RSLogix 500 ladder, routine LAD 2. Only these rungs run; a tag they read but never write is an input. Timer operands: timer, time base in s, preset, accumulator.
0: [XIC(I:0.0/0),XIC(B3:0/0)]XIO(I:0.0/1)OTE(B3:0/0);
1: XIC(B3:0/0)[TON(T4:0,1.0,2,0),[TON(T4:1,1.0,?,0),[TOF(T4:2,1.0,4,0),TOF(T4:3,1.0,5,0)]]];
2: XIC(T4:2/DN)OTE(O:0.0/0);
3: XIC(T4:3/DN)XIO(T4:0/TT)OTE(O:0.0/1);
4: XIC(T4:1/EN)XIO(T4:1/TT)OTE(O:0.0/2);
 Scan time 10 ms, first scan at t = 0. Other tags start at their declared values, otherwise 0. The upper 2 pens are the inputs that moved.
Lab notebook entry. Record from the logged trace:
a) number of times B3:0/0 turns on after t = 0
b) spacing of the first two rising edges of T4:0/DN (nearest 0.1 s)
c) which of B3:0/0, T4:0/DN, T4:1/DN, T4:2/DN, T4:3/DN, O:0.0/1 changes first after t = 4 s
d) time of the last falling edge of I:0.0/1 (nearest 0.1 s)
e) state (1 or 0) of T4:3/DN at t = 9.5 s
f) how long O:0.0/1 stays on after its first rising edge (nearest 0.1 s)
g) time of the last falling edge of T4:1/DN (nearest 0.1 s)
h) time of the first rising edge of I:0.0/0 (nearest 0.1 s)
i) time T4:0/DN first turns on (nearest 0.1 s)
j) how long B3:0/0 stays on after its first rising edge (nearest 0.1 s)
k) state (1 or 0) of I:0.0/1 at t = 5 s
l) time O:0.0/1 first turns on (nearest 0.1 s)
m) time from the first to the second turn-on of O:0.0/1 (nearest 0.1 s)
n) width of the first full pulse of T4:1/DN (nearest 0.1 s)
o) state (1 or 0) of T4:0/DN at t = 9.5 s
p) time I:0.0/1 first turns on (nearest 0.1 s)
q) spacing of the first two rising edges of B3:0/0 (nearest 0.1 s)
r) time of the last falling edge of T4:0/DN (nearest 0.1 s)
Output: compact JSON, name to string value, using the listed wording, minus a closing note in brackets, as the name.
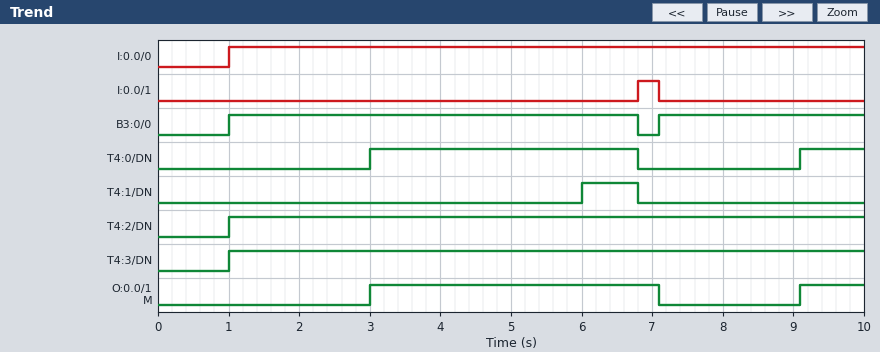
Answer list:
{"number of times B3:0/0 turns on after t = 0": "2", "spacing of the first two rising edges of T4:0/DN": "6.1 s", "which of B3:0/0, T4:0/DN, T4:1/DN, T4:2/DN, T4:3/DN, O:0.0/1 changes first after t = 4 s": "T4:1/DN", "time of the last falling edge of I:0.0/1": "7.1 s", "state (1 or 0) of T4:3/DN at t = 9.5 s": "1", "how long O:0.0/1 stays on after its first rising edge": "4.1 s", "time of the last falling edge of T4:1/DN": "6.8 s", "time of the first rising edge of I:0.0/0": "1.0 s", "time T4:0/DN first turns on": "3.0 s", "how long B3:0/0 stays on after its first rising edge": "5.8 s", "state (1 or 0) of I:0.0/1 at t = 5 s": "0", "time O:0.0/1 first turns on": "3.0 s", "time from the first to the second turn-on of O:0.0/1": "6.1 s", "width of the first full pulse of T4:1/DN": "0.8 s", "state (1 or 0) of T4:0/DN at t = 9.5 s": "1", "time I:0.0/1 first turns on": "6.8 s", "spacing of the first two rising edges of B3:0/0": "6.1 s", "time of the last falling edge of T4:0/DN": "6.8 s"}
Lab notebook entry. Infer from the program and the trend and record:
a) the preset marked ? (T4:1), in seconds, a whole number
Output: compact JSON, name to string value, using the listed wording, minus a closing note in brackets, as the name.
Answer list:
{"the preset marked ? (T4:1), in seconds, a whole number": "5 s"}
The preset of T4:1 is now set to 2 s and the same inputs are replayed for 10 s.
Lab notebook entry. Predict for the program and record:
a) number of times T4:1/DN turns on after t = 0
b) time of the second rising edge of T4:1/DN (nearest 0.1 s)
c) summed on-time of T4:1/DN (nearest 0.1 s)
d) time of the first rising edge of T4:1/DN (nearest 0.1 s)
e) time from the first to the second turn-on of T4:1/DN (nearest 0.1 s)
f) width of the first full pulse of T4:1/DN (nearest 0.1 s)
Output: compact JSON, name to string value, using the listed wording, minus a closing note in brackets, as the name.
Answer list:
{"number of times T4:1/DN turns on after t = 0": "2", "time of the second rising edge of T4:1/DN": "9.1 s", "summed on-time of T4:1/DN": "4.7 s", "time of the first rising edge of T4:1/DN": "3.0 s", "time from the first to the second turn-on of T4:1/DN": "6.1 s", "width of the first full pulse of T4:1/DN": "3.8 s"}
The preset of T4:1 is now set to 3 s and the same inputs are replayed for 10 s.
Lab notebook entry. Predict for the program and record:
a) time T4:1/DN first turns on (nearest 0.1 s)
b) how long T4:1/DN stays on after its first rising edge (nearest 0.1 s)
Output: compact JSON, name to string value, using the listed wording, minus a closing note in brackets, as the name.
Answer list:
{"time T4:1/DN first turns on": "4.0 s", "how long T4:1/DN stays on after its first rising edge": "2.8 s"}
